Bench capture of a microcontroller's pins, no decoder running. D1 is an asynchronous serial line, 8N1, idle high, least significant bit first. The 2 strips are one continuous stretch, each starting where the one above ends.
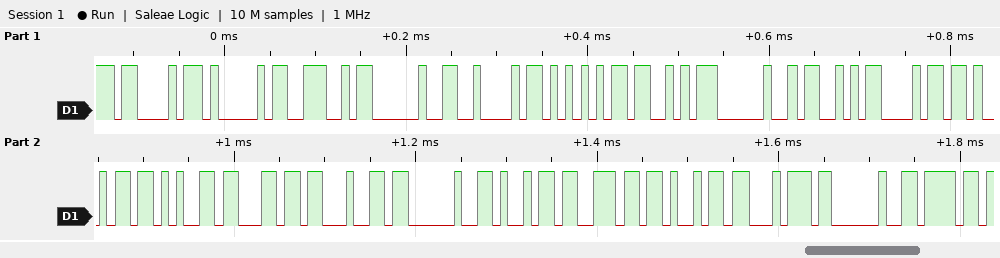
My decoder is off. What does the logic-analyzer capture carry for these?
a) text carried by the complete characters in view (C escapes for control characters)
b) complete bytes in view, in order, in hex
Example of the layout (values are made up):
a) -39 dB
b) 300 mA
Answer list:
a) "CAN BUS Shield init o"
b) 43 41 4E 20 42 55 53 20 53 68 69 65 6C 64 20 69 6E 69 74 20 6F
